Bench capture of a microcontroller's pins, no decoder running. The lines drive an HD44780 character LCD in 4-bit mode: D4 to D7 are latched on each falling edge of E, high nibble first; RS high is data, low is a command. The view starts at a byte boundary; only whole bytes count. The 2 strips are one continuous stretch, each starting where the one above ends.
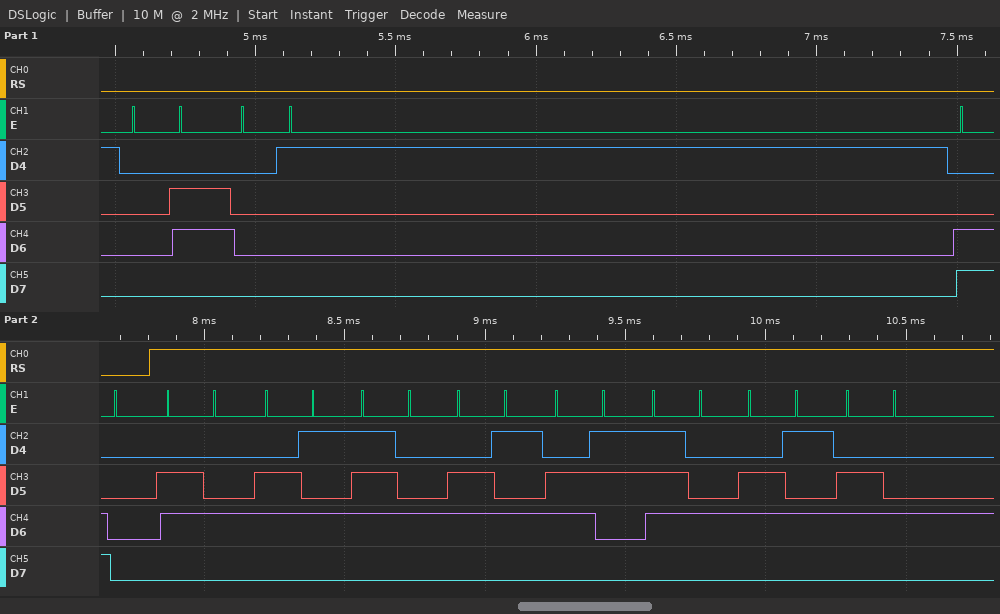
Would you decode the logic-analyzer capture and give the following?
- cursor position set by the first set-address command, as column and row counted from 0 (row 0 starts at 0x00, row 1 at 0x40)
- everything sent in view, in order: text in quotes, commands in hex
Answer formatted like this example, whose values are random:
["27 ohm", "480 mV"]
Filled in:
["column 0, row 1", "0x06 0x01 0xC0 \"detected\""]
